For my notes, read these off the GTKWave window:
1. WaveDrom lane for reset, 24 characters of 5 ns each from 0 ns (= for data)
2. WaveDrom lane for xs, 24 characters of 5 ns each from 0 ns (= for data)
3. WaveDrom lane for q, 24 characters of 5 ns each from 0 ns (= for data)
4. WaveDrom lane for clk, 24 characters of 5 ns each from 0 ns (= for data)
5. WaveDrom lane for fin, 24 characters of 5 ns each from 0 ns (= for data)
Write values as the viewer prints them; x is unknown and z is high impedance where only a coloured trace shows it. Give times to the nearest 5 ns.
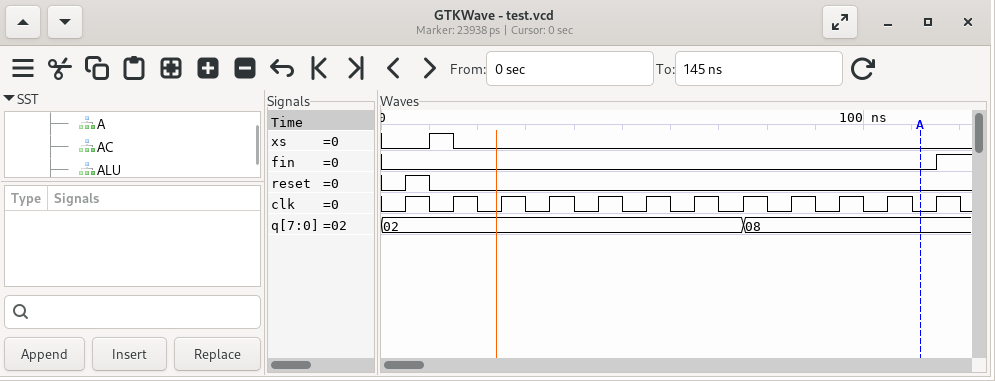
{name: 'reset', wave: '010.....................'}
{name: 'xs', wave: '0.10....................'}
{name: 'q', wave: '=..............=........', data: '02 08'}
{name: 'clk', wave: '010101010101010101010101'}
{name: 'fin', wave: '0......................1'}
